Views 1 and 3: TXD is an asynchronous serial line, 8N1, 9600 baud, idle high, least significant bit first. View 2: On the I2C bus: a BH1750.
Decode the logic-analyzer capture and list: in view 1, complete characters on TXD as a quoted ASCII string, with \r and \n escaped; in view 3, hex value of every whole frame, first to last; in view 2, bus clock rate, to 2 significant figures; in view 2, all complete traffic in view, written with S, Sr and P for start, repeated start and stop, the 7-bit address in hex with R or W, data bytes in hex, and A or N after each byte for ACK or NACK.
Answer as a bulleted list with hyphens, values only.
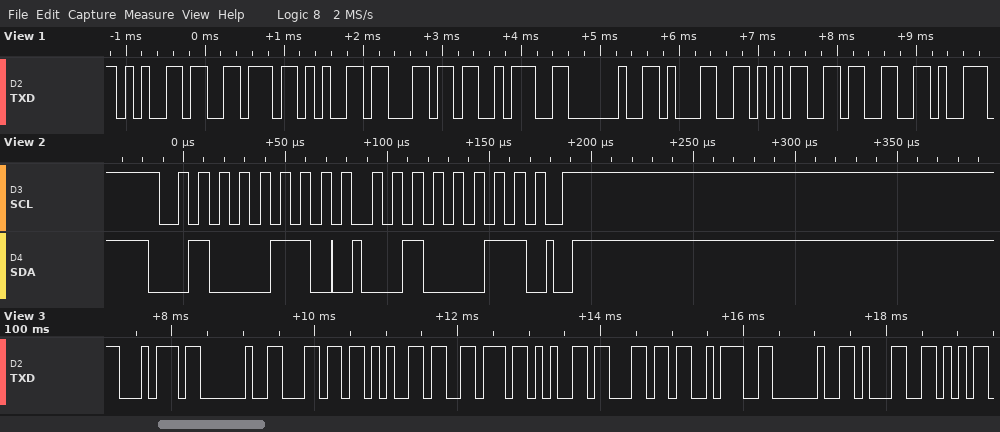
- "evel: 153"
- 0x74 0x20 0x6C 0x65 0x76 0x65 0x6C 0x3A 0x20 0x31
- 100 kHz
- S 23W A 23 A P
